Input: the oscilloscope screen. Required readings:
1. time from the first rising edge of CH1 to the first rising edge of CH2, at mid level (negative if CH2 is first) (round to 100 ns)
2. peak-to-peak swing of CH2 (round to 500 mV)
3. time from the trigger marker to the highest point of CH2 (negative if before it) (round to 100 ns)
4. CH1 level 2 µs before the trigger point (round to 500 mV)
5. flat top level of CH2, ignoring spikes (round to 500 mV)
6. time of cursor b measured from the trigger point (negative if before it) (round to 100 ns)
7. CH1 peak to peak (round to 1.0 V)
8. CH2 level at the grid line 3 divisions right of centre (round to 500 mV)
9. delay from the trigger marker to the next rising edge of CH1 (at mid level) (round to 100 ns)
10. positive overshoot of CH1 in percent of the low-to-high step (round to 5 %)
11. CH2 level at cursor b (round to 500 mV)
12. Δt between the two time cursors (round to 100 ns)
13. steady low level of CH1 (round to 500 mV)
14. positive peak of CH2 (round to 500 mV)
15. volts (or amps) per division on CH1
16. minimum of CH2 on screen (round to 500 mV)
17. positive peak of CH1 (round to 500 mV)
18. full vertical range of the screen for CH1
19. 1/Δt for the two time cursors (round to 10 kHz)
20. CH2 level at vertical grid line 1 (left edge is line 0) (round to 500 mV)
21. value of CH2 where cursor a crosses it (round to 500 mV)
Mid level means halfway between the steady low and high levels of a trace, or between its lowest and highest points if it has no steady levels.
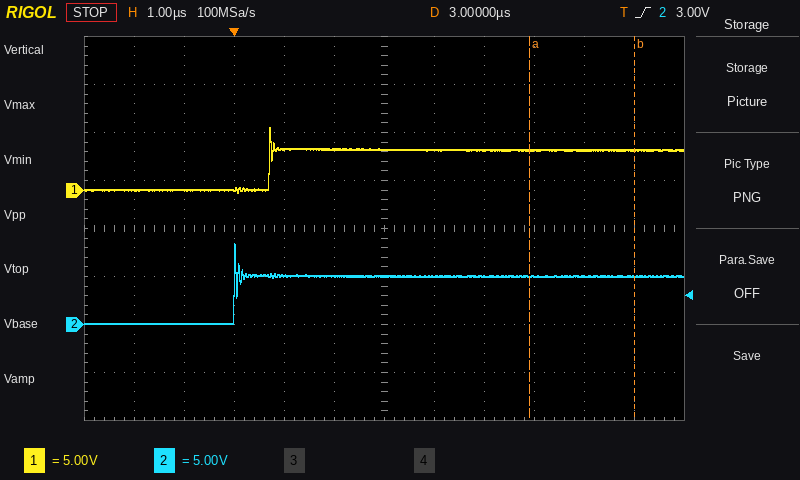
-700 ns
8.5 V
0.0 µs
0.0 V
5.0 V
+8.0 µs
7.0 V
5.0 V
700 ns
55 %
5.0 V
2.1 µs
0.0 V
8.5 V
5 V
0.0 V
6.5 V
40 V
480 kHz
0.0 V
5.0 V
